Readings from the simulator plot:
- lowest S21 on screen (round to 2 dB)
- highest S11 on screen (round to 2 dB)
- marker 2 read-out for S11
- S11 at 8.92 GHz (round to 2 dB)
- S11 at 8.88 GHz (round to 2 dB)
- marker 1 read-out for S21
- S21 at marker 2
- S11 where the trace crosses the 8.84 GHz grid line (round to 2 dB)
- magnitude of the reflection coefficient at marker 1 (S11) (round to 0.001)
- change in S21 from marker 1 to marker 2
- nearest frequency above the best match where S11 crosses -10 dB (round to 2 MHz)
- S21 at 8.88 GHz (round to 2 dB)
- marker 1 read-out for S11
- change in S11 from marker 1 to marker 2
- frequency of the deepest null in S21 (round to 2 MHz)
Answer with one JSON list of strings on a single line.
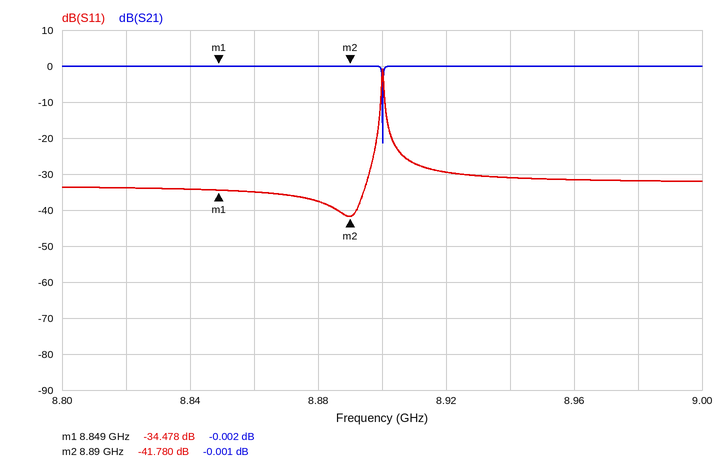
["-22 dB", "0 dB", "-41.780 dB", "-30 dB", "-38 dB", "-0.002 dB", "-0.001 dB", "-34 dB", "0.019", "0.001 dB", "8.900 GHz", "0 dB", "-34.478 dB", "-7.302 dB", "8.900 GHz"]
